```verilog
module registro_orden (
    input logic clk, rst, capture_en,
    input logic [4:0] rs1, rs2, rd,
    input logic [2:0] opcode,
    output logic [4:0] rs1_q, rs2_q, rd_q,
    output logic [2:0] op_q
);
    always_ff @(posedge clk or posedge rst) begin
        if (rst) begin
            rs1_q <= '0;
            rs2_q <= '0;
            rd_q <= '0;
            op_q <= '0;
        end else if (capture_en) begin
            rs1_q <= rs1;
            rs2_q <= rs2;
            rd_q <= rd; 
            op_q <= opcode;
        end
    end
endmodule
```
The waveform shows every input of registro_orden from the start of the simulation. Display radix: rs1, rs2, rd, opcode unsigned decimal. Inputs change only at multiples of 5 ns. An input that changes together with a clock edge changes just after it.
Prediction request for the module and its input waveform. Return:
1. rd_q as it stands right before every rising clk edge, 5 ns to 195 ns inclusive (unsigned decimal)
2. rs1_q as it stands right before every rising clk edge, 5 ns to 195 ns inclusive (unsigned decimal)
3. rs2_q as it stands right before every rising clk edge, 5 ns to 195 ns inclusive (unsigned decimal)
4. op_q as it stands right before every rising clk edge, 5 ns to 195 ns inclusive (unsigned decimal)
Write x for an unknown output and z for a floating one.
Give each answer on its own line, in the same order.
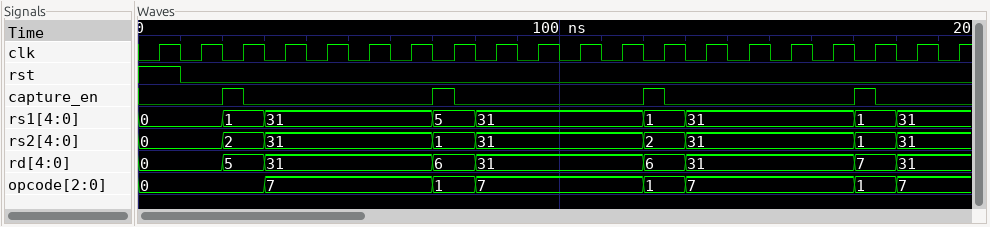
0, 0, 0, 5, 5, 5, 5, 5, 6, 6, 6, 6, 6, 6, 6, 6, 6, 6, 7, 7
0, 0, 0, 1, 1, 1, 1, 1, 5, 5, 5, 5, 5, 1, 1, 1, 1, 1, 1, 1
0, 0, 0, 2, 2, 2, 2, 2, 1, 1, 1, 1, 1, 2, 2, 2, 2, 2, 1, 1
0, 0, 0, 0, 0, 0, 0, 0, 1, 1, 1, 1, 1, 1, 1, 1, 1, 1, 1, 1
